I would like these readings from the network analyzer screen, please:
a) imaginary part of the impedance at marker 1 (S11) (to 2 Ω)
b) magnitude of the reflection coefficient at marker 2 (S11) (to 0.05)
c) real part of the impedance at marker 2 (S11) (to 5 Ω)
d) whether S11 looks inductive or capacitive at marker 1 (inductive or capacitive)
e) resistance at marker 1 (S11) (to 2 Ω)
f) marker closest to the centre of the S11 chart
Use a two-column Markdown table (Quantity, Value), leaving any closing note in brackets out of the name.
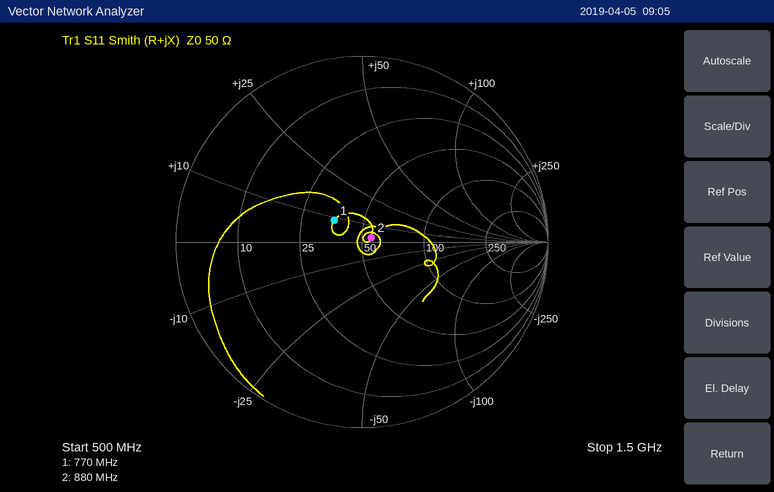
| Quantity | Value |
|---|---|
| imaginary part of the impedance at marker 1 (S11) | +8 Ω |
| magnitude of the reflection coefficient at marker 2 (S11) | 0.05 |
| real part of the impedance at marker 2 (S11) | 55 Ω |
| whether S11 looks inductive or capacitive at marker 1 | inductive |
| resistance at marker 1 (S11) | 36 Ω |
| marker closest to the centre of the S11 chart | marker 2 |
